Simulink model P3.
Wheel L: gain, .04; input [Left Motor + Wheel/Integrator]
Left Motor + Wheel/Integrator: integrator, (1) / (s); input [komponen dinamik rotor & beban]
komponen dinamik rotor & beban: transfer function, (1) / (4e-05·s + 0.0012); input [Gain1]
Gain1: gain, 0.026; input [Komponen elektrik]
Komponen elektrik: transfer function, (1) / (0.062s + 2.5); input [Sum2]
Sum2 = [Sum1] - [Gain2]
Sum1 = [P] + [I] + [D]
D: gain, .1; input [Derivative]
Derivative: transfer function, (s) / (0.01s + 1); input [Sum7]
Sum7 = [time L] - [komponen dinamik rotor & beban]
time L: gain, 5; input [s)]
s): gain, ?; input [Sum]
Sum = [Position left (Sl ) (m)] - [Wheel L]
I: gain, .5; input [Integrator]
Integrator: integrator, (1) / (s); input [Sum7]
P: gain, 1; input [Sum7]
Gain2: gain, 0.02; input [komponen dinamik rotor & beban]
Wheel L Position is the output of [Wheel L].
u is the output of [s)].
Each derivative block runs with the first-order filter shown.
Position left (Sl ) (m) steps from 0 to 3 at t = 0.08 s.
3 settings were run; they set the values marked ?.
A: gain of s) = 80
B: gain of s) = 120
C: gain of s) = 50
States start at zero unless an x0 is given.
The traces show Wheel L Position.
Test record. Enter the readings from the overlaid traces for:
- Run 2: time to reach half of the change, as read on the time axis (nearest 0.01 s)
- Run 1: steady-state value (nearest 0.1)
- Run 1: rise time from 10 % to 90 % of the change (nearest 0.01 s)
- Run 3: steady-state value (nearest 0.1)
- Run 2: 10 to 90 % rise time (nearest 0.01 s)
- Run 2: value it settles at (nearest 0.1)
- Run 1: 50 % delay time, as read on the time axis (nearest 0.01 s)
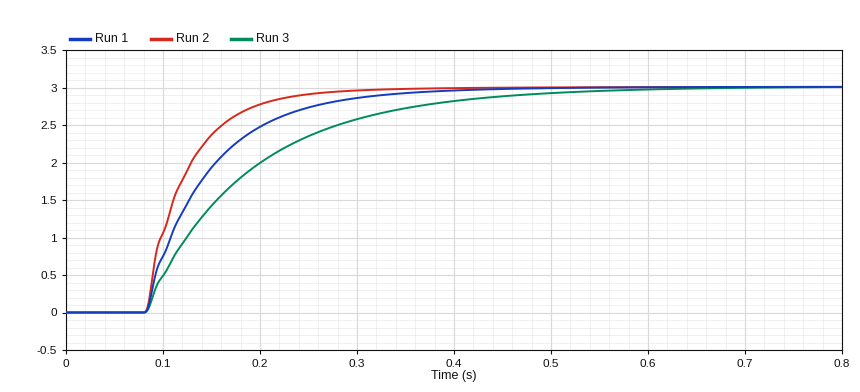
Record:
0.11 s
3.0
0.15 s
3.0
0.10 s
3.0
0.13 s
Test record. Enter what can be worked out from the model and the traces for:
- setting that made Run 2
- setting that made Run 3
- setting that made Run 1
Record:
B
C
A
